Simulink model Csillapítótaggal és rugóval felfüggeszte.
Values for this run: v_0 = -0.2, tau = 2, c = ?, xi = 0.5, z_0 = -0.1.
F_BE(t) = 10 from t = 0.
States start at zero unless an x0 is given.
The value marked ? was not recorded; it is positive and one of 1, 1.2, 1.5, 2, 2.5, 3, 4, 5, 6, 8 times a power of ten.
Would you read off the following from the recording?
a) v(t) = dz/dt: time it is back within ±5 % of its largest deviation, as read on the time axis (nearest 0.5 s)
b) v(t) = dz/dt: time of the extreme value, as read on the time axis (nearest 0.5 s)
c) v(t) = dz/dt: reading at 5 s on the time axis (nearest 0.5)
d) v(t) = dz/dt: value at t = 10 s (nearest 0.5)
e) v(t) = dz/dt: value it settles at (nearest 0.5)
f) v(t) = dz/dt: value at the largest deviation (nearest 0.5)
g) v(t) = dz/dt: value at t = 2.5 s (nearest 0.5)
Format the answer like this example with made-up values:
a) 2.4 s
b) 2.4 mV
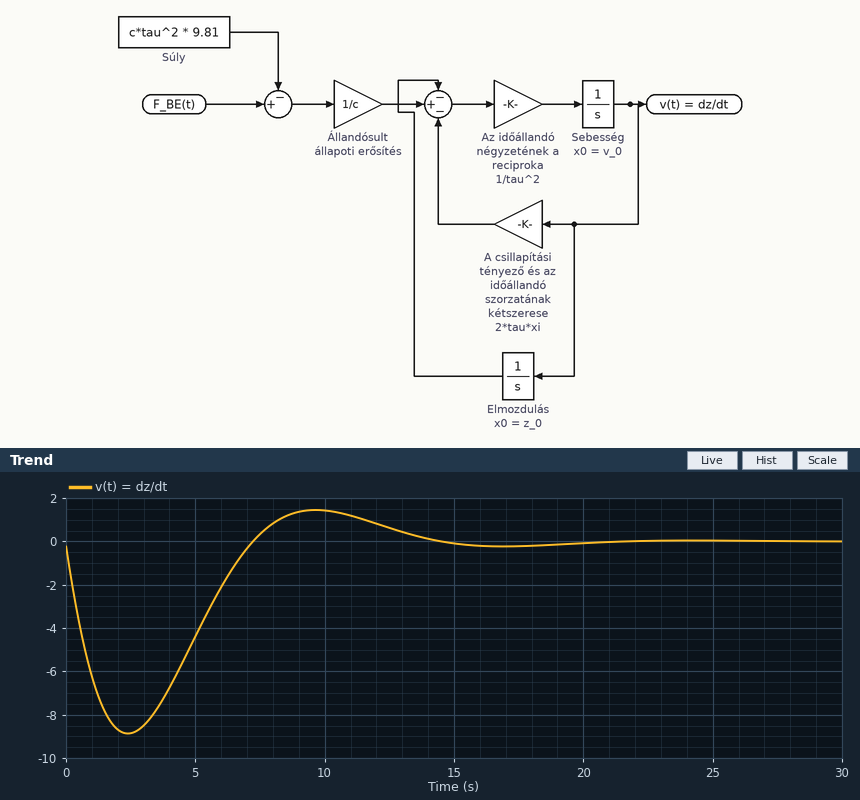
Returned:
a) 13.0 s
b) 2.5 s
c) -4.5
d) 1.5
e) 0.0
f) -9.0
g) -9.0
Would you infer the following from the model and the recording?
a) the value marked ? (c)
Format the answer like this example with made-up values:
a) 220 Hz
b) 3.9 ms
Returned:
a) 1.5
